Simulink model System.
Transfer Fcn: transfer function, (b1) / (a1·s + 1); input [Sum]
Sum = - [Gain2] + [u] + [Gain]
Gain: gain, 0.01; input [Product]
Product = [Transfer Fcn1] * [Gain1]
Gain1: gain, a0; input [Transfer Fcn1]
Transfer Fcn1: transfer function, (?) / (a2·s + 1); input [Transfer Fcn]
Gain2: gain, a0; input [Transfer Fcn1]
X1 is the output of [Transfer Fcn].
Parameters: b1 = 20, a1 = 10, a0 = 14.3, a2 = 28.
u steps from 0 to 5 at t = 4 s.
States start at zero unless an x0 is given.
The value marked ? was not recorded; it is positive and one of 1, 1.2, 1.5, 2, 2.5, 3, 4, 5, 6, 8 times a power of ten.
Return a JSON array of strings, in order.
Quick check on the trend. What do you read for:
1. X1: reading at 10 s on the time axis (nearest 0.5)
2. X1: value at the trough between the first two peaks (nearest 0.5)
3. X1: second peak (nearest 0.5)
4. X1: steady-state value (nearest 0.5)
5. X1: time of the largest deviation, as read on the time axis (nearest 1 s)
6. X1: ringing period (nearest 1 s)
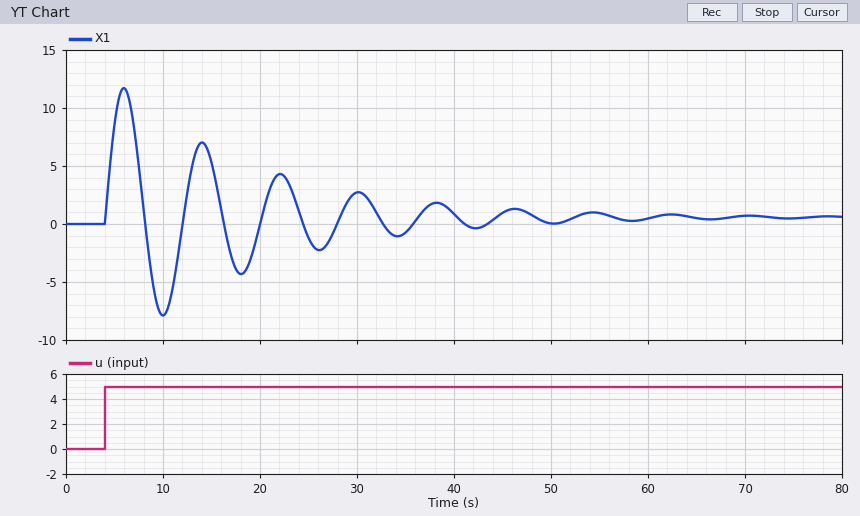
["-8.0", "-8.0", "7.0", "0.5", "6 s", "8 s"]
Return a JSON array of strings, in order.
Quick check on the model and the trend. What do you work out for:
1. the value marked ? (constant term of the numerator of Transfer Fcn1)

["0.6"]
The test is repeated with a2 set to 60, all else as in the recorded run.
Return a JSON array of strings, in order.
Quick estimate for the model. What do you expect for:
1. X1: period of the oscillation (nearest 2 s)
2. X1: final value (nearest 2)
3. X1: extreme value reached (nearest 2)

["12 s", "0", "16"]
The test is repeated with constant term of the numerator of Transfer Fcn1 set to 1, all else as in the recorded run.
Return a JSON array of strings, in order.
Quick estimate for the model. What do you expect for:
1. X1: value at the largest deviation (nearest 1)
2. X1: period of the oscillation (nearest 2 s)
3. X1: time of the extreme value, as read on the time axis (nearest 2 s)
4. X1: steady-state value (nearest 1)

["9", "6 s", "6 s", "0"]
